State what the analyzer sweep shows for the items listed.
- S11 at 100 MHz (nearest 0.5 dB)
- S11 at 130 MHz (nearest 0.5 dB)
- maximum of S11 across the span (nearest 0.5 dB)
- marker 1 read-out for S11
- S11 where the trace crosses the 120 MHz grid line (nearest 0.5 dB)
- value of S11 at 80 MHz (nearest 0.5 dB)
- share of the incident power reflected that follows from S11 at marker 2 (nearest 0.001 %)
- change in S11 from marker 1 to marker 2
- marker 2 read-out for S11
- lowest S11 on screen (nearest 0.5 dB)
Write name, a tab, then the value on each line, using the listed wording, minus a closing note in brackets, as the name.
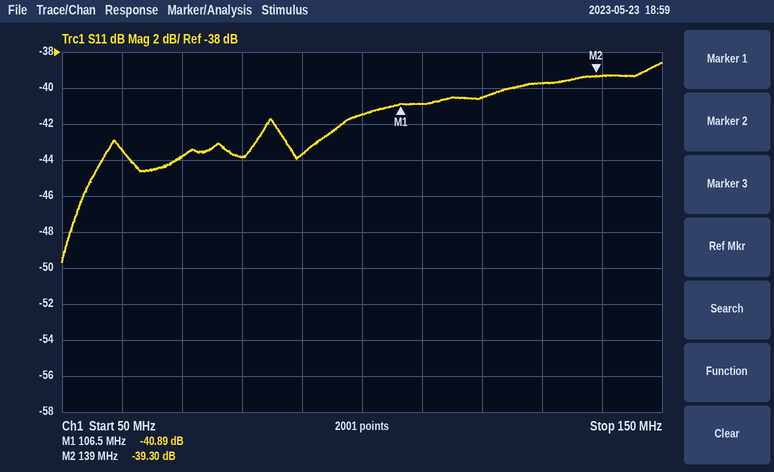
S11 at 100 MHz	-41.5 dB
S11 at 130 MHz	-39.5 dB
maximum of S11 across the span	-38.5 dB
marker 1 read-out for S11	-40.89 dB
S11 where the trace crosses the 120 MHz grid line	-40.5 dB
value of S11 at 80 MHz	-44.0 dB
share of the incident power reflected that follows from S11 at marker 2	0.012 %
change in S11 from marker 1 to marker 2	1.59 dB
marker 2 read-out for S11	-39.30 dB
lowest S11 on screen	-49.5 dB
